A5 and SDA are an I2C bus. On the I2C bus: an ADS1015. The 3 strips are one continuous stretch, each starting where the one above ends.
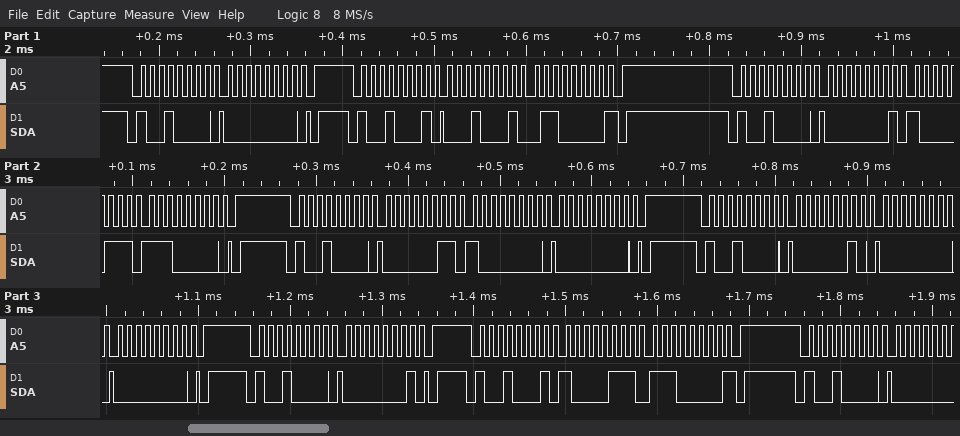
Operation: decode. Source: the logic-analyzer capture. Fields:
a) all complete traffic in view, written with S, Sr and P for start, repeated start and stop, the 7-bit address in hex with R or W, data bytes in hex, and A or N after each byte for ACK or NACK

S 48W A 00 A P S 48R A 11 A 60 N P S 48W A 01 A 87 A E0 A P S 48W A 03 A 80 A 00 A P S 48W A 02 A 00 A 00 A P S 48W A 01 A P S 48R A 87 A E0 N P S 48W A
